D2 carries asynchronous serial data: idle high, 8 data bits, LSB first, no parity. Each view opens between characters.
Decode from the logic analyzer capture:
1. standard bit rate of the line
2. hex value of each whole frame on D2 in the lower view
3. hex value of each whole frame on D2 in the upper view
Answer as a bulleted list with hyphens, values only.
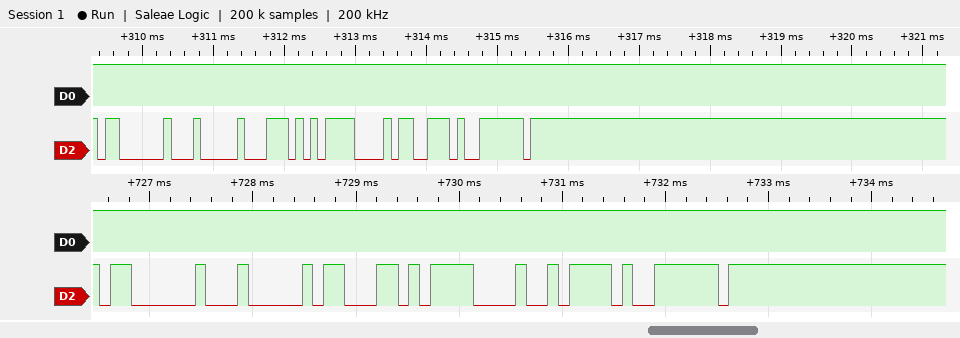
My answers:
- 9600 baud
- 03, 04, 63, 0F, 7A, 7E
- 03, 04, 5C, 0F, 73, 7E
